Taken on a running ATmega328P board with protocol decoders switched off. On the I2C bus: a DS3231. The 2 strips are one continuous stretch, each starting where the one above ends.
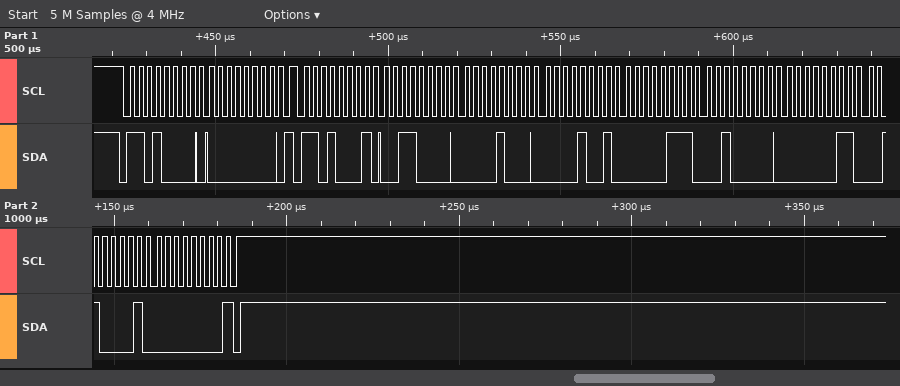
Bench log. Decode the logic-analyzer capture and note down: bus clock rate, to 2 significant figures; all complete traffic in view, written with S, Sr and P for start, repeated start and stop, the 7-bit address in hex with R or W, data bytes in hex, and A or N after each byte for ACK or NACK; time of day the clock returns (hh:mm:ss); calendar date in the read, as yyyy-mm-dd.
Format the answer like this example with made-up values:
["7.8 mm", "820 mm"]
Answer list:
["400 kHz", "S 68W A 00 A Sr 68R A 30 A 08 A 09 A 07 A 20 A 03 A 21 A 00 N P", "09:08:30", "2021-03-20"]
